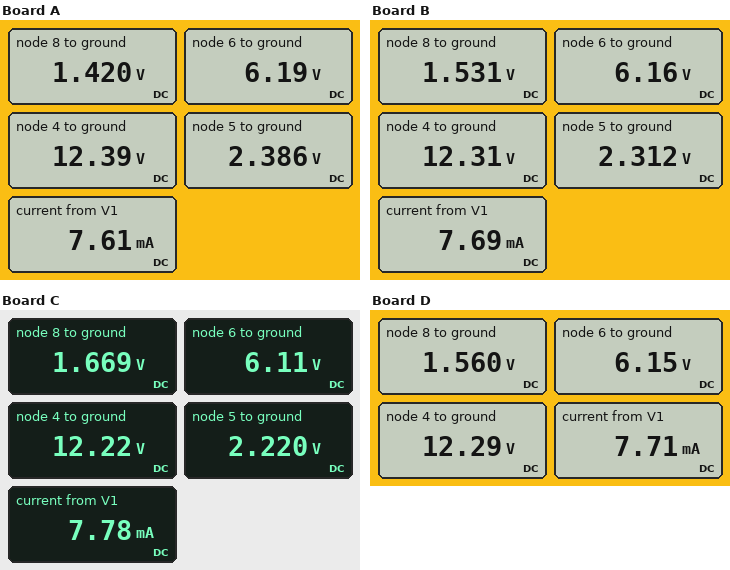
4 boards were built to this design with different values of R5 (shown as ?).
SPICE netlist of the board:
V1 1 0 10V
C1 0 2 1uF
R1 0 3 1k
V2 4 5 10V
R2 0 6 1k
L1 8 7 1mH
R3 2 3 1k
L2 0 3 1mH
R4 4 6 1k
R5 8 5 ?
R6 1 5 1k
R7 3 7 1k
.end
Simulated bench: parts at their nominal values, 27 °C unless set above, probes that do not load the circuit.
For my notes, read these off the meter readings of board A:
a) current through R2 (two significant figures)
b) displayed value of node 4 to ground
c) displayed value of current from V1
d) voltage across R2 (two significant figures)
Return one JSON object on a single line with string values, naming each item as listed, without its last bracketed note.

{"current through R2": "6.2 mA", "displayed value of node 4 to ground": "12.39 V", "displayed value of current from V1": "7.61 mA", "voltage across R2": "6.2 V"}
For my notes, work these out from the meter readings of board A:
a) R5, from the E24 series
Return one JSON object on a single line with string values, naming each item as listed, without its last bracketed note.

{"R5, from the E24 series": "680 Ω"}
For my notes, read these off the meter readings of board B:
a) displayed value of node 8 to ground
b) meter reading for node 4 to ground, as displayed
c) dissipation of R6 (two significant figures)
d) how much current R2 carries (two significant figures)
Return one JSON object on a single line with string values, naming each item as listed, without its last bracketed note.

{"displayed value of node 8 to ground": "1.531 V", "meter reading for node 4 to ground, as displayed": "12.31 V", "dissipation of R6": "59 mW", "how much current R2 carries": "6.2 mA"}
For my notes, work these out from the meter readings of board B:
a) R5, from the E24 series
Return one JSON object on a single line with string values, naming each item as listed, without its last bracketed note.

{"R5, from the E24 series": "510 Ω"}
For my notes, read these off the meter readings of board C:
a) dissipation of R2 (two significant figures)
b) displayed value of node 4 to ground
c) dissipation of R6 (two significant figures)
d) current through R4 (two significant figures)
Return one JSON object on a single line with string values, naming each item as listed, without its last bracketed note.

{"dissipation of R2": "37 mW", "displayed value of node 4 to ground": "12.22 V", "dissipation of R6": "61 mW", "current through R4": "6.1 mA"}
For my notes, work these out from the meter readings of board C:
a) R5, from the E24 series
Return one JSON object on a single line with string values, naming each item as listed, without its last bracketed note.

{"R5, from the E24 series": "330 Ω"}
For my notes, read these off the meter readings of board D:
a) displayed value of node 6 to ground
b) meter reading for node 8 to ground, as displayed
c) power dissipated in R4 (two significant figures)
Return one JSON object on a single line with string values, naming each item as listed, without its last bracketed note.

{"displayed value of node 6 to ground": "6.15 V", "meter reading for node 8 to ground, as displayed": "1.560 V", "power dissipated in R4": "38 mW"}
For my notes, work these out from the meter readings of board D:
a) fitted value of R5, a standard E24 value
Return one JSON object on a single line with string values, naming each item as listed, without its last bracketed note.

{"fitted value of R5, a standard E24 value": "470 Ω"}
